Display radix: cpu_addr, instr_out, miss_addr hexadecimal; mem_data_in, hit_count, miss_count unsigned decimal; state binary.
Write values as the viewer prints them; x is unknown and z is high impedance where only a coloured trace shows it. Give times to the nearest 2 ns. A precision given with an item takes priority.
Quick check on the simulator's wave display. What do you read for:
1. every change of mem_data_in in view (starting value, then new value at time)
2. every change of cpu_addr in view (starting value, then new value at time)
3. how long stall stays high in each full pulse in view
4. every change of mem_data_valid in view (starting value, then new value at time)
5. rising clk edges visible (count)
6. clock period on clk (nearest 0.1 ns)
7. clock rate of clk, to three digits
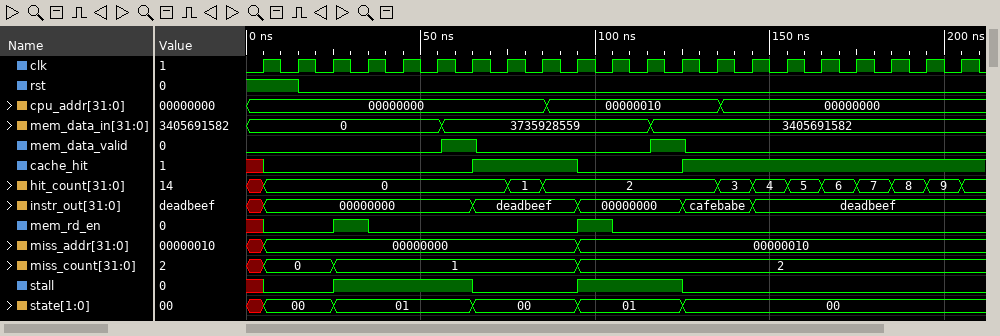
0, 3735928559 at 56 ns, 3405691582 at 116 ns
00000000, 00000010 at 86 ns, 00000000 at 136 ns
40 ns, 30 ns
0, 1 at 56 ns, 0 at 66 ns, 1 at 116 ns, 0 at 126 ns
21
10 ns
100 MHz
